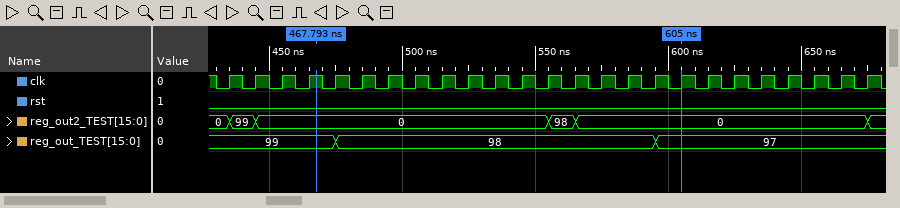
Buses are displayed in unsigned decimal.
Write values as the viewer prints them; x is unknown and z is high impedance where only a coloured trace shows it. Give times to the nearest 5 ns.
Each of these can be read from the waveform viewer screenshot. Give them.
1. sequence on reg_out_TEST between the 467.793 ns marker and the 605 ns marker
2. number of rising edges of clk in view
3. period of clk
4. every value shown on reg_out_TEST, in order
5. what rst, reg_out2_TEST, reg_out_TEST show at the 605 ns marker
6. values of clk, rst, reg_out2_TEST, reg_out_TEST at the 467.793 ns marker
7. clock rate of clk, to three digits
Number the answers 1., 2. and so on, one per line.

1. 99, 98, 97
2. 25
3. 10 ns
4. 99, 98, 97
5. rst=0, reg_out2_TEST=0, reg_out_TEST=97
6. clk=1, rst=0, reg_out2_TEST=0, reg_out_TEST=99
7. 100 MHz
